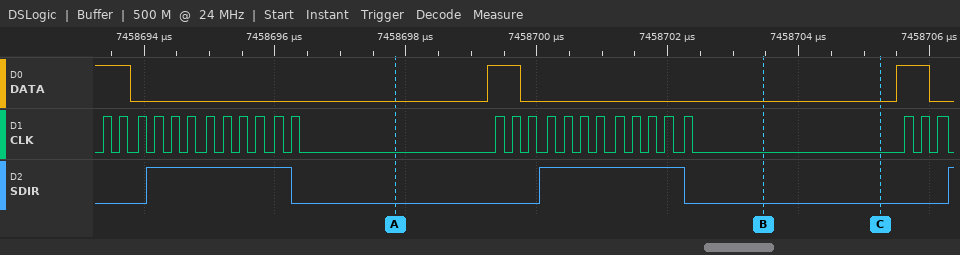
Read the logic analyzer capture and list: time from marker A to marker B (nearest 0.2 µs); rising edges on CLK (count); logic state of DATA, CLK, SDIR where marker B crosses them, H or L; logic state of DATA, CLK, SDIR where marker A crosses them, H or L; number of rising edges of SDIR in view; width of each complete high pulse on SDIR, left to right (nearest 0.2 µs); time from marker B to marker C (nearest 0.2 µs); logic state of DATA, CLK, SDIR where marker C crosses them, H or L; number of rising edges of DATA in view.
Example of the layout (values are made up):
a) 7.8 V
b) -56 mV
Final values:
a) 5.6 µs
b) 27
c) DATA=L, CLK=L, SDIR=L
d) DATA=L, CLK=L, SDIR=L
e) 3
f) 2.2 µs, 2.2 µs
g) 1.8 µs
h) DATA=L, CLK=L, SDIR=L
i) 2
